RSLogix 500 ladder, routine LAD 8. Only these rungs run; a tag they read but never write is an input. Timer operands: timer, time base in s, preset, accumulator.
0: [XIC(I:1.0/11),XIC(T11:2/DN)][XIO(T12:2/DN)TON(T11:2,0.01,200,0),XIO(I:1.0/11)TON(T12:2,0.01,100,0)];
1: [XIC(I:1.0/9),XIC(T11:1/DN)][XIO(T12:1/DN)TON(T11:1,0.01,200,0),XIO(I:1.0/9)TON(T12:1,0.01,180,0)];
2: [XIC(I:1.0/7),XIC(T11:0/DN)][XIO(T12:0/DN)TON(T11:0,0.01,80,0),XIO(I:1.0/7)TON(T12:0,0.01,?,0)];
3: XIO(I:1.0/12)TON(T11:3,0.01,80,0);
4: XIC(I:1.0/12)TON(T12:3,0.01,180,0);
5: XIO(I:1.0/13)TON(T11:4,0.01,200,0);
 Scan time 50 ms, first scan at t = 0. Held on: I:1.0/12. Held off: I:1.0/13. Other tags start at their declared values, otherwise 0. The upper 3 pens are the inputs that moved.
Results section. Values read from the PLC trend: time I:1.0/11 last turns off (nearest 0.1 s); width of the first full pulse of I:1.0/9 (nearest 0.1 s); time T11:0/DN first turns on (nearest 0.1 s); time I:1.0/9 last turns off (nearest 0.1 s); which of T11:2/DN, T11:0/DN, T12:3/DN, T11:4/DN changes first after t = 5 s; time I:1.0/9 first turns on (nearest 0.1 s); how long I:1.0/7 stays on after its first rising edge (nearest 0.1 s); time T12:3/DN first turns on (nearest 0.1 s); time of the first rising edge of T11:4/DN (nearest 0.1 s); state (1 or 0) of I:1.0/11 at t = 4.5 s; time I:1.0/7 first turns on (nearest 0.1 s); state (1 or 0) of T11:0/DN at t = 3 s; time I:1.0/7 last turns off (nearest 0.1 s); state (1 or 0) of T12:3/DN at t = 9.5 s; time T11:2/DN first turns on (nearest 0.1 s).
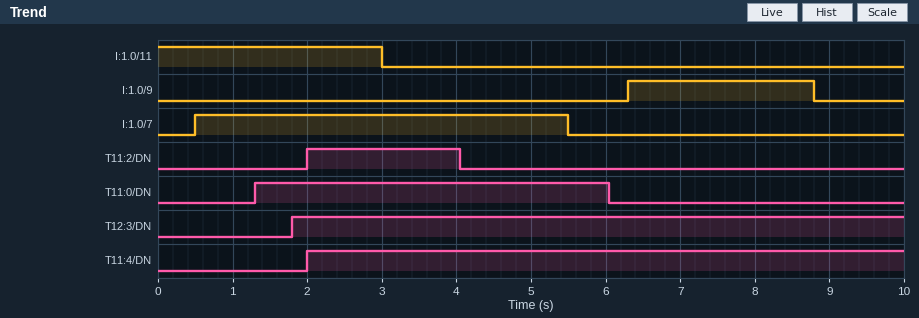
3.0 s
2.5 s
1.3 s
8.8 s
T11:0/DN
6.3 s
5.0 s
1.8 s
2.0 s
0
0.5 s
1
5.5 s
1
2.0 s
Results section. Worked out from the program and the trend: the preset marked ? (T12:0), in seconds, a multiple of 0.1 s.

0.5 s
